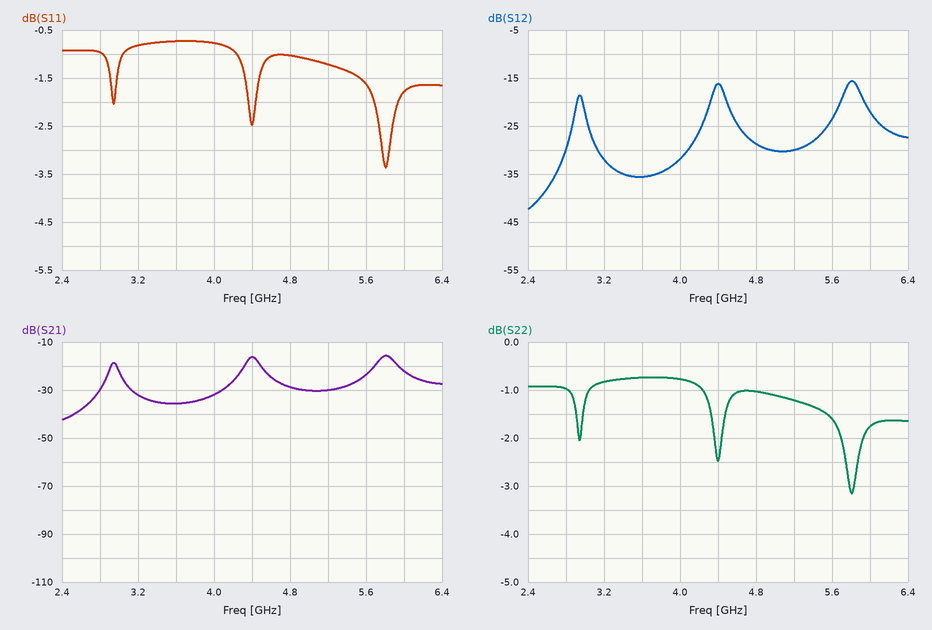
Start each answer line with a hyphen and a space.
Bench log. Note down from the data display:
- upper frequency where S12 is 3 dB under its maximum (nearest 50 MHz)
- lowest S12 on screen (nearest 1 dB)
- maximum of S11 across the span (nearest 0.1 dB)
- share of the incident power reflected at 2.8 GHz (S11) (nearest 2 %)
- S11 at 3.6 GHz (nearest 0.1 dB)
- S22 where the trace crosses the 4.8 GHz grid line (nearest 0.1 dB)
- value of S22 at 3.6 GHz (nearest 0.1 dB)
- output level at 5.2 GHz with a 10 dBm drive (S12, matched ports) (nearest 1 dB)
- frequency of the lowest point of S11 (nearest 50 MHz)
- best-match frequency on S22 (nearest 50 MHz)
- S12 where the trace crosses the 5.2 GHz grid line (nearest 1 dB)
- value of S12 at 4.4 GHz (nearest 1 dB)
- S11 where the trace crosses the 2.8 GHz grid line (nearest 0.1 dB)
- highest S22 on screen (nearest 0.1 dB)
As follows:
- 5.90 GHz
- -42 dB
- -0.7 dB
- 80 %
- -0.7 dB
- -1.0 dB
- -0.7 dB
- -20 dBm
- 5.80 GHz
- 5.80 GHz
- -30 dB
- -16 dB
- -1.0 dB
- -0.7 dB
